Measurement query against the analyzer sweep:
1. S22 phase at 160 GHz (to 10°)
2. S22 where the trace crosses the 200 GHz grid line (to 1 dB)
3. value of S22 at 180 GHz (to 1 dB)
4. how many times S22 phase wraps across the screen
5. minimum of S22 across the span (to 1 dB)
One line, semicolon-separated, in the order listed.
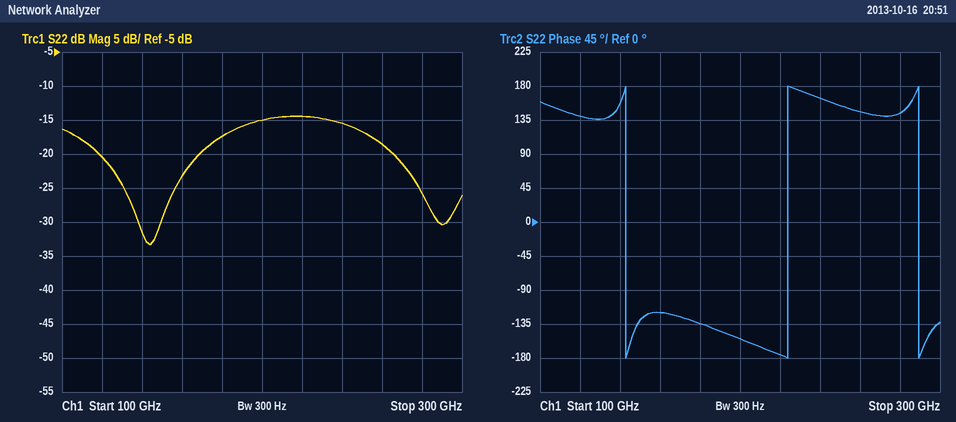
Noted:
-120°; -15 dB; -17 dB; 3; -33 dB
